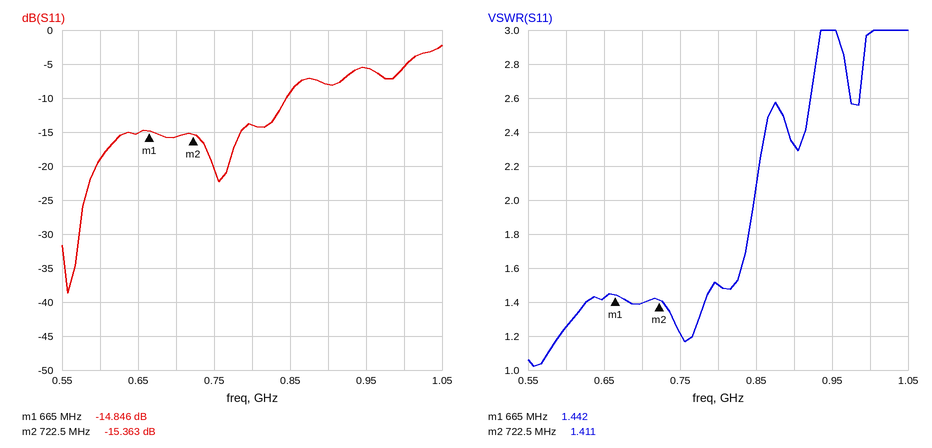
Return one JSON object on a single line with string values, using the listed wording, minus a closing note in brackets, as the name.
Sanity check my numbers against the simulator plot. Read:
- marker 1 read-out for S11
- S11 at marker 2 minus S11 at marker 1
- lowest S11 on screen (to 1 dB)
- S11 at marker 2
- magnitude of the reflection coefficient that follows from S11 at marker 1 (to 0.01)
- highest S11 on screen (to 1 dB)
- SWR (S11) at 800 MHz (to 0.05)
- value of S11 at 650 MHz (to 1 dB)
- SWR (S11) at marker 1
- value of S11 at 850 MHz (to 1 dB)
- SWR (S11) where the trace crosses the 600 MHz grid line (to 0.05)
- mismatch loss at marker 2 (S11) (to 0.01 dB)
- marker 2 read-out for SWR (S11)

{"marker 1 read-out for S11": "-14.846 dB", "S11 at marker 2 minus S11 at marker 1": "-0.517 dB", "lowest S11 on screen": "-39 dB", "S11 at marker 2": "-15.363 dB", "magnitude of the reflection coefficient that follows from S11 at marker 1": "0.18", "highest S11 on screen": "-2 dB", "SWR (S11) at 800 MHz": "1.50", "value of S11 at 650 MHz": "-15 dB", "SWR (S11) at marker 1": "1.442", "value of S11 at 850 MHz": "-9 dB", "SWR (S11) where the trace crosses the 600 MHz grid line": "1.25", "mismatch loss at marker 2 (S11)": "0.13 dB", "marker 2 read-out for SWR": "1.411"}
